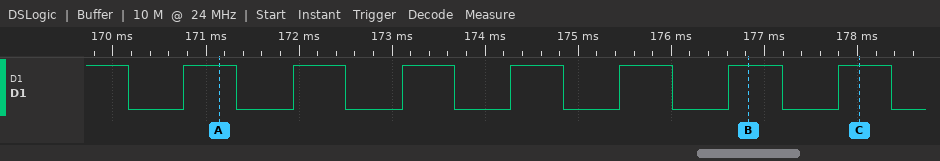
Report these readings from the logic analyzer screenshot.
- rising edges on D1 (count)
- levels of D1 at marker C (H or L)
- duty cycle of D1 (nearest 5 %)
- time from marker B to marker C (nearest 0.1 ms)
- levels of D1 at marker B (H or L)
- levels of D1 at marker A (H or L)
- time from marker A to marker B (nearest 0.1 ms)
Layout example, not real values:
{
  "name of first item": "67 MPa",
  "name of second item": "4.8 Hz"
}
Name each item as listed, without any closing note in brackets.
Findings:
{
  "rising edges on D1": "7",
  "levels of D1 at marker C": "D1=H",
  "duty cycle of D1": "50 %",
  "time from marker B to marker C": "1.2 ms",
  "levels of D1 at marker B": "D1=H",
  "levels of D1 at marker A": "D1=H",
  "time from marker A to marker B": "5.7 ms"
}
